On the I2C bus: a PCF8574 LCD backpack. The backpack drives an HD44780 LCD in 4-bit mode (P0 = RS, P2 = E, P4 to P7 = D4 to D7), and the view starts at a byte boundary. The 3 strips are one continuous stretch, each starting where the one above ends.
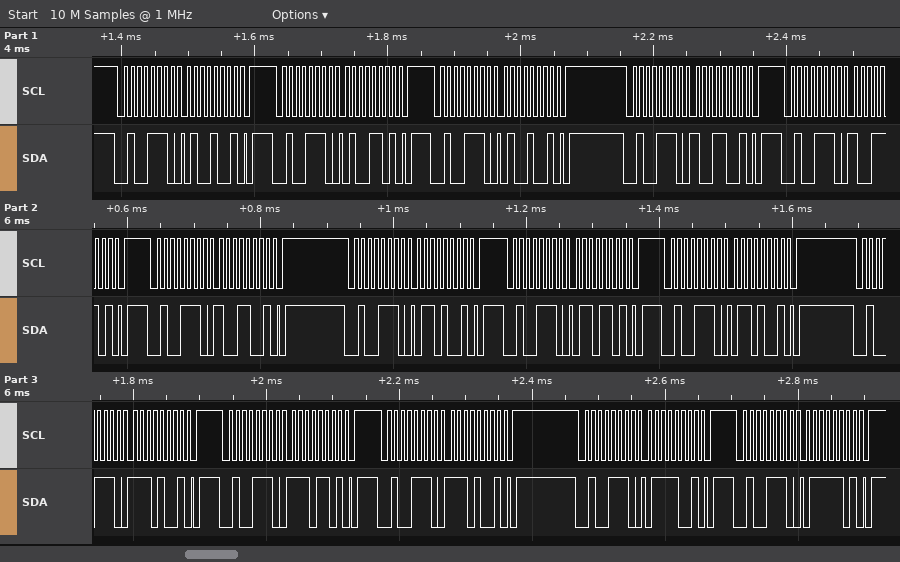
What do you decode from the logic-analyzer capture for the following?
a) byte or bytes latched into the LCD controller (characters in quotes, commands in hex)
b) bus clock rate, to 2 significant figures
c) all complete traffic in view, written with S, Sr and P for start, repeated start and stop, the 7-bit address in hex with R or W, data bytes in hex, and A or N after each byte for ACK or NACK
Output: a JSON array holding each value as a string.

["'I' 'n'", "100 kHz", "S 27W A 49 A P S 27W A 4D A P S 27W A 49 A P S 27W A 99 A P S 27W A 9D A P S 27W A 99 A P S 27W A 69 A P S 27W A 6D A P S 27W A 69 A P S 27W A E9 A P S 27W A ED A P S 27W A E9 A P S 27W A 79 A P S 27W A 7D A P"]
